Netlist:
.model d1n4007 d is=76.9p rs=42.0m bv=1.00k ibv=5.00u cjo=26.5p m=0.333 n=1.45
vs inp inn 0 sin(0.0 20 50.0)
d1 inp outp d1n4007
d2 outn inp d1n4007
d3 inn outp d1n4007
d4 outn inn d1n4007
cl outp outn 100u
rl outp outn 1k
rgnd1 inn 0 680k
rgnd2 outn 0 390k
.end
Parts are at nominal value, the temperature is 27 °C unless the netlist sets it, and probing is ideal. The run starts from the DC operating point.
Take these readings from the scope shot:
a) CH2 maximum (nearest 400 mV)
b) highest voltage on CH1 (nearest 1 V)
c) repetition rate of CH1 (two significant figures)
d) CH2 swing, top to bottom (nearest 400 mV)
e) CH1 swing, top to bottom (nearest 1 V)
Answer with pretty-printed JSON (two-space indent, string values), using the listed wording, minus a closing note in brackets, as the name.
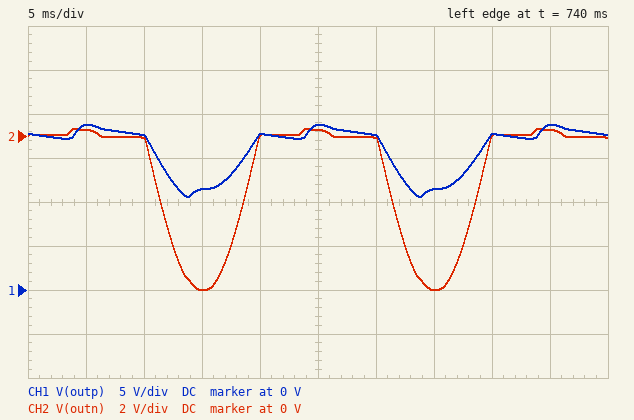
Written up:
{
  "CH2 maximum": "400 mV",
  "highest voltage on CH1": "19 V",
  "repetition rate of CH1": "50 Hz",
  "CH2 swing, top to bottom": "7.2 V",
  "CH1 swing, top to bottom": "8 V"
}
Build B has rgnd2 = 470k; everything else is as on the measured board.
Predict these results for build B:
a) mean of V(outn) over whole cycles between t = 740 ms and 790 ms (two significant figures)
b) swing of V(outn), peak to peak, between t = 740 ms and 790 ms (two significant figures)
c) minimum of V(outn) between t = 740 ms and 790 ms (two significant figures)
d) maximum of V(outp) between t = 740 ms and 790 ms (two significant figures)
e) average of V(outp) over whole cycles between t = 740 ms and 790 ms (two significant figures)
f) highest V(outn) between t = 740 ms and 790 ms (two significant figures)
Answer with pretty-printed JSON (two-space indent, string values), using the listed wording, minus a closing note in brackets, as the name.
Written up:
{
  "mean of V(outn) over whole cycles between t = 740 ms and 790 ms": "-2.5 V",
  "swing of V(outn), peak to peak, between t = 740 ms and 790 ms": "8.2 V",
  "minimum of V(outn) between t = 740 ms and 790 ms": "-7.9 V",
  "maximum of V(outp) between t = 740 ms and 790 ms": "19 V",
  "average of V(outp) over whole cycles between t = 740 ms and 790 ms": "15 V",
  "highest V(outn) between t = 740 ms and 790 ms": "340 mV"
}
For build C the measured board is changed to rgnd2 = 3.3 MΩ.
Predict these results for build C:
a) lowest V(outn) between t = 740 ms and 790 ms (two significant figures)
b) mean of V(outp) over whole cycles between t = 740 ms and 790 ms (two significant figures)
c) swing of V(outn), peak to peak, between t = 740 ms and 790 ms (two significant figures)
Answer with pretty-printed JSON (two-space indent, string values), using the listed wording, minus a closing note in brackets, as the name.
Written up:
{
  "lowest V(outn) between t = 740 ms and 790 ms": "-16 V",
  "mean of V(outp) over whole cycles between t = 740 ms and 790 ms": "13 V",
  "swing of V(outn), peak to peak, between t = 740 ms and 790 ms": "17 V"
}
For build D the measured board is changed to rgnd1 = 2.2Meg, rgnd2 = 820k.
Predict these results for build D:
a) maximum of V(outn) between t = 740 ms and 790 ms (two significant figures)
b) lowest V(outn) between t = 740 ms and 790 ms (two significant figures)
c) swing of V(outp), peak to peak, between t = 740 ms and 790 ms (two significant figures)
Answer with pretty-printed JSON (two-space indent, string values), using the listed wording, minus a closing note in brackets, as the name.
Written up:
{
  "maximum of V(outn) between t = 740 ms and 790 ms": "220 mV",
  "lowest V(outn) between t = 740 ms and 790 ms": "-5.2 V",
  "swing of V(outp), peak to peak, between t = 740 ms and 790 ms": "6.5 V"
}
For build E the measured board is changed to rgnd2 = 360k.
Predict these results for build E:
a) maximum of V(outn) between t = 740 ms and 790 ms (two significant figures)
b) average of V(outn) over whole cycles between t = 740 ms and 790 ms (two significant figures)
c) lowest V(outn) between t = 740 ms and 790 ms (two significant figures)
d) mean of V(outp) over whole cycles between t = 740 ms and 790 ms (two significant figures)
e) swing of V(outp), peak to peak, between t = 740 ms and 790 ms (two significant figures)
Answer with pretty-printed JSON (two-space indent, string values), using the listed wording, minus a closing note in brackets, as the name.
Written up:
{
  "maximum of V(outn) between t = 740 ms and 790 ms": "290 mV",
  "average of V(outn) over whole cycles between t = 740 ms and 790 ms": "-2.1 V",
  "lowest V(outn) between t = 740 ms and 790 ms": "-6.7 V",
  "mean of V(outp) over whole cycles between t = 740 ms and 790 ms": "16 V",
  "swing of V(outp), peak to peak, between t = 740 ms and 790 ms": "7.9 V"
}
